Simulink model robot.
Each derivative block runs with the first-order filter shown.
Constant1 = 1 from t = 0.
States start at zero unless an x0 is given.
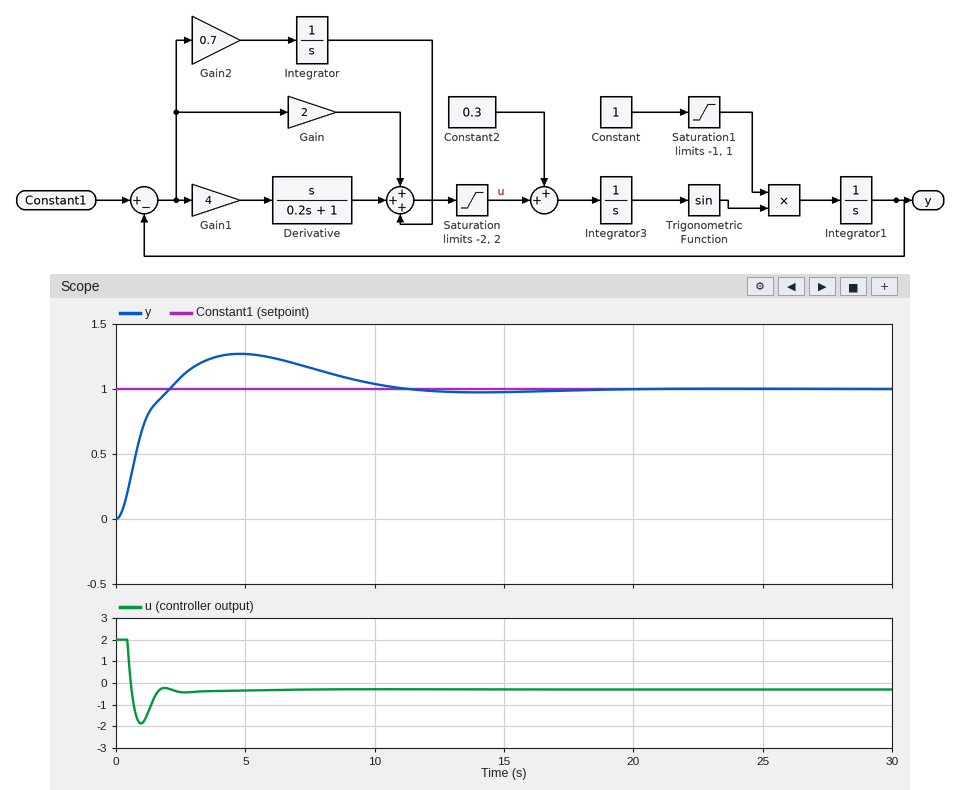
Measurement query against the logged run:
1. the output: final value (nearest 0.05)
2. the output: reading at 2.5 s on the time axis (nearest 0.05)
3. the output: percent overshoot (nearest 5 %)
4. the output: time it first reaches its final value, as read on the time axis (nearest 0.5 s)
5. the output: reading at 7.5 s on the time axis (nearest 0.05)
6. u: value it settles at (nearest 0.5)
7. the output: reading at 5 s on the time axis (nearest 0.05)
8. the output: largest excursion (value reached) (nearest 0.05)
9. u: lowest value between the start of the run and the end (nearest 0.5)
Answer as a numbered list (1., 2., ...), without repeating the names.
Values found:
1. 1.00
2. 1.10
3. 25 %
4. 2.0 s
5. 1.15
6. -0.5
7. 1.25
8. 1.25
9. -2.0
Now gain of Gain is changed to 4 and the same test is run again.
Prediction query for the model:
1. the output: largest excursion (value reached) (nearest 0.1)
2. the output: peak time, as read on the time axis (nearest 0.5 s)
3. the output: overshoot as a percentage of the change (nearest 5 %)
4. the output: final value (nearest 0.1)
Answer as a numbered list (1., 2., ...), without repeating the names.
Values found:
1. 1.2
2. 3.5 s
3. 15 %
4. 1.0
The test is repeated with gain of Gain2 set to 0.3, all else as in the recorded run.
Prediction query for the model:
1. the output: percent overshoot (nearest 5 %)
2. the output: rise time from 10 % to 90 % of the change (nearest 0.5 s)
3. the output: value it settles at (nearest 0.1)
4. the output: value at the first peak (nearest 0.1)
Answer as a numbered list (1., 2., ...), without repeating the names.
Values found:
1. 20 %
2. 1.5 s
3. 1.0
4. 1.2
